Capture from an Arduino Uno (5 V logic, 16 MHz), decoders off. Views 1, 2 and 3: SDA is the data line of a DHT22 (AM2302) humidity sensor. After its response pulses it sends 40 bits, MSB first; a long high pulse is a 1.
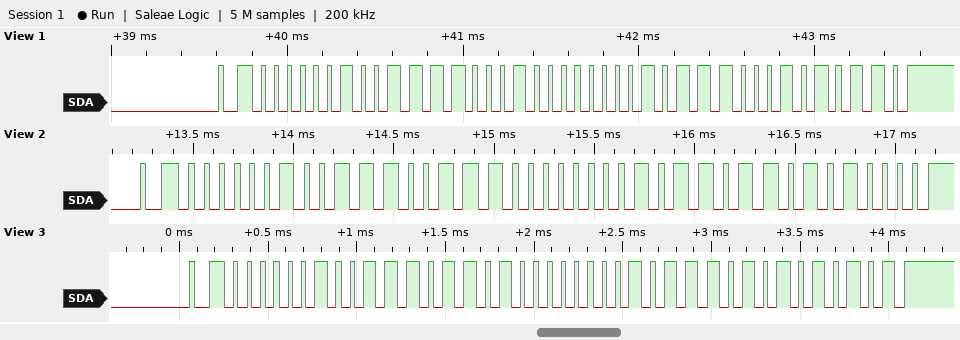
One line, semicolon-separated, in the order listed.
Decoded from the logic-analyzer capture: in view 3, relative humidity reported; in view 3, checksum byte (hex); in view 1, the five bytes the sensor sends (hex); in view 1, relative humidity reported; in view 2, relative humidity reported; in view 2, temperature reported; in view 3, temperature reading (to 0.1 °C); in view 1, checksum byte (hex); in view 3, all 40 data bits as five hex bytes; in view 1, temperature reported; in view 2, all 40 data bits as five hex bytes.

63.0 %; 0x55; 02 78 80 5C 56; 63.2 %; 62.7 %; -9.1 °C; -9.3 °C; 0x56; 02 76 80 5D 55; -9.2 °C; 02 73 80 5B 50
